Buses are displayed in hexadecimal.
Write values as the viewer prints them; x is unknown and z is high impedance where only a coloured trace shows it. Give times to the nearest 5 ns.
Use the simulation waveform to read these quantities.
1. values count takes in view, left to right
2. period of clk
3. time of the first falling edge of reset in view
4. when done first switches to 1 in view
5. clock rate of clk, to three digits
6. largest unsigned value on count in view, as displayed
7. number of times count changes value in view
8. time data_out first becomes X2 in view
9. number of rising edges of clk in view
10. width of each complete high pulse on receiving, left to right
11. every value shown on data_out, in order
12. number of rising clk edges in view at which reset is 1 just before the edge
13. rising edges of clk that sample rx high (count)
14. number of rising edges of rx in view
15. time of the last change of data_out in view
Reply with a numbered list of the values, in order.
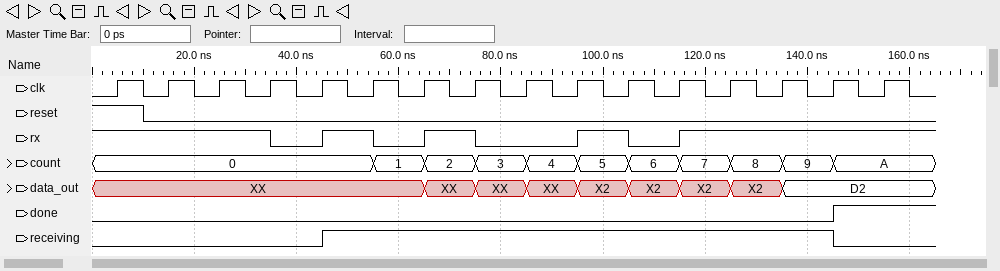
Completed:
1. 0, 1, 2, 3, 4, 5, 6, 7, 8, 9, A
2. 10 ns
3. 10 ns
4. 145 ns
5. 100 MHz
6. A
7. 10
8. 95 ns
9. 16
10. 100 ns
11. XX, XX, XX, XX, X2, X2, X2, X2, D2
12. 1
13. 11
14. 4
15. 135 ns
